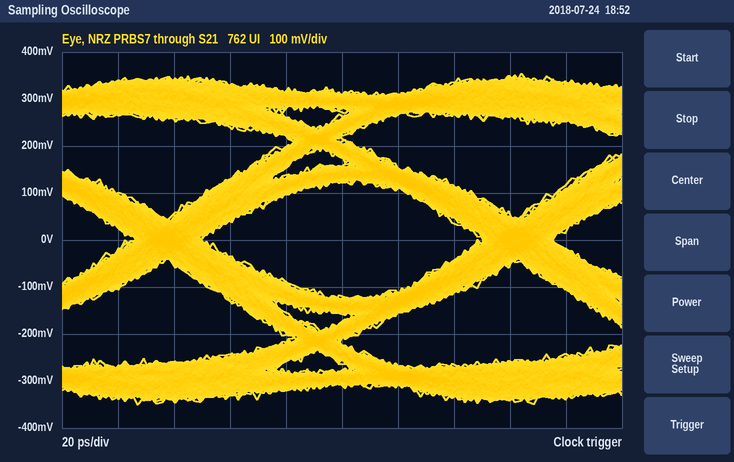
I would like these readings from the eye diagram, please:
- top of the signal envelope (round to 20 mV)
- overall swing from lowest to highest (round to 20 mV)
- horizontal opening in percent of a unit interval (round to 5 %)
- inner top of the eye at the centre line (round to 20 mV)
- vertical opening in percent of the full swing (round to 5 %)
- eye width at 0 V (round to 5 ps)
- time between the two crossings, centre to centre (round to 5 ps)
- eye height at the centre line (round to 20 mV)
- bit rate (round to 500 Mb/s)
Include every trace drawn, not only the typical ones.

360 mV
700 mV
80 %
120 mV
35 %
100 ps
125 ps
240 mV
8.0 Gb/s
